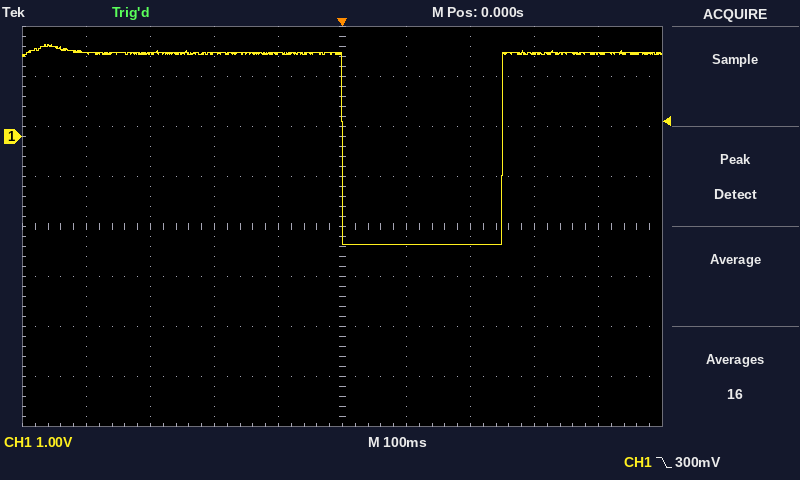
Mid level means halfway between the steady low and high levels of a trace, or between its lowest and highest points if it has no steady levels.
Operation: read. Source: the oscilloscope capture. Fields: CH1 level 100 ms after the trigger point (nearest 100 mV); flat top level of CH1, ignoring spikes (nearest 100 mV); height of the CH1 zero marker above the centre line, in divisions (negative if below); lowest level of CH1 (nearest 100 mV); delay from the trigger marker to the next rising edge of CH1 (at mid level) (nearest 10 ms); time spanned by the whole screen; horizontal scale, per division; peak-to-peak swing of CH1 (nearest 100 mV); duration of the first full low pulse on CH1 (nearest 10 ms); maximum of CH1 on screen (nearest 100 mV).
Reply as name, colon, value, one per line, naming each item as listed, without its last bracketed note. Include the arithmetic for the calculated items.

CH1 level 100 ms after the trigger point: -2.2 V
flat top level of CH1, ignoring spikes: 1.7 V
height of the CH1 zero marker above the centre line, in divisions: +1.8 div
lowest level of CH1: -2.2 V
delay from the trigger marker to the next rising edge of CH1 (at mid level): 250 ms
time spanned by the whole screen: 1 s
horizontal scale, per division: 100 ms
peak-to-peak swing of CH1: 1.8 V − (-2.2 V) = 4.0 V
duration of the first full low pulse on CH1: 250 ms
maximum of CH1 on screen: 1.8 V
